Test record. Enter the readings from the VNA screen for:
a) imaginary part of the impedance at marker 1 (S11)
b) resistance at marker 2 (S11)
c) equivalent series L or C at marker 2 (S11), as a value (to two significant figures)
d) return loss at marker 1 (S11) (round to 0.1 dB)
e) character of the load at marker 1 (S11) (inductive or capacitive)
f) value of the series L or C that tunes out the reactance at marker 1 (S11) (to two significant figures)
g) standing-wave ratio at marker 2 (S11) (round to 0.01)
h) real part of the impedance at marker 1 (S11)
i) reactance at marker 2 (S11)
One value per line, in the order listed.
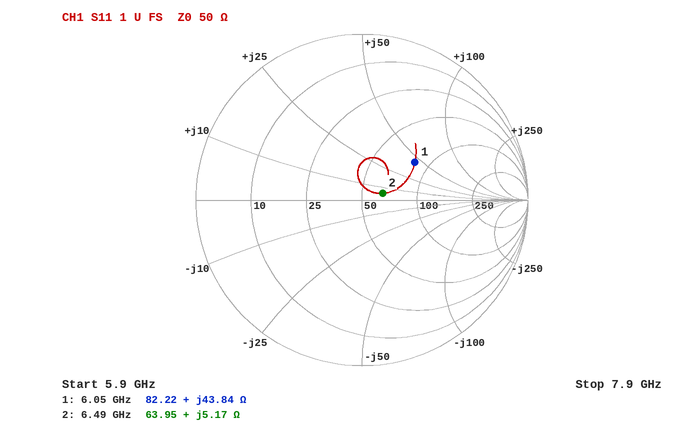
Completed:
+43.84 Ω
63.95 Ω
130 pH
8.2 dB
inductive
600 fF
1.30
82.22 Ω
+5.17 Ω
